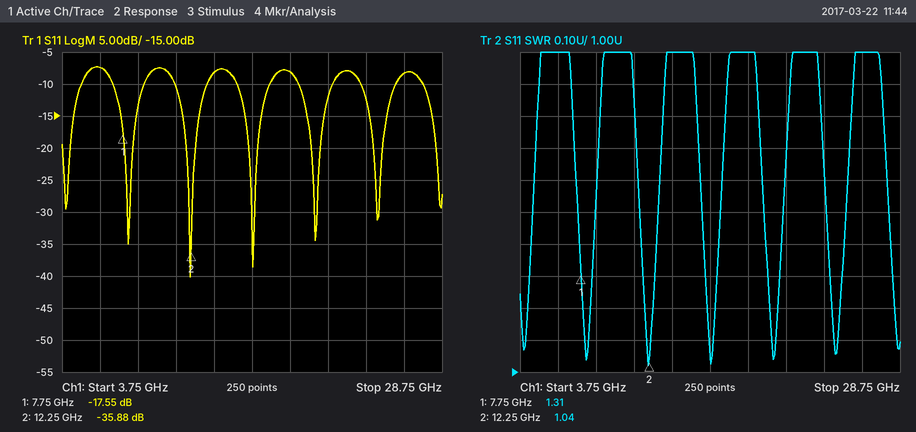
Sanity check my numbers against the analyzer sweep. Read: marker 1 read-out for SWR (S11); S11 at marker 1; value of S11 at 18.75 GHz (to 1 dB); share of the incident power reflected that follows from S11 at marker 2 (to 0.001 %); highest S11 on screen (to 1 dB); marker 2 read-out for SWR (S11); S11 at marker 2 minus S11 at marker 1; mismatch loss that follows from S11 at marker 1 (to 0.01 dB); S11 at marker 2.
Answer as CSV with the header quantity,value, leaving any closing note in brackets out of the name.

quantity,value
marker 1 read-out for SWR,1.31
S11 at marker 1,-17.55 dB
value of S11 at 18.75 GHz,-8 dB
share of the incident power reflected that follows from S11 at marker 2,0.026 %
highest S11 on screen,-7 dB
marker 2 read-out for SWR,1.04
S11 at marker 2 minus S11 at marker 1,-18.33 dB
mismatch loss that follows from S11 at marker 1,0.08 dB
S11 at marker 2,-35.88 dB
